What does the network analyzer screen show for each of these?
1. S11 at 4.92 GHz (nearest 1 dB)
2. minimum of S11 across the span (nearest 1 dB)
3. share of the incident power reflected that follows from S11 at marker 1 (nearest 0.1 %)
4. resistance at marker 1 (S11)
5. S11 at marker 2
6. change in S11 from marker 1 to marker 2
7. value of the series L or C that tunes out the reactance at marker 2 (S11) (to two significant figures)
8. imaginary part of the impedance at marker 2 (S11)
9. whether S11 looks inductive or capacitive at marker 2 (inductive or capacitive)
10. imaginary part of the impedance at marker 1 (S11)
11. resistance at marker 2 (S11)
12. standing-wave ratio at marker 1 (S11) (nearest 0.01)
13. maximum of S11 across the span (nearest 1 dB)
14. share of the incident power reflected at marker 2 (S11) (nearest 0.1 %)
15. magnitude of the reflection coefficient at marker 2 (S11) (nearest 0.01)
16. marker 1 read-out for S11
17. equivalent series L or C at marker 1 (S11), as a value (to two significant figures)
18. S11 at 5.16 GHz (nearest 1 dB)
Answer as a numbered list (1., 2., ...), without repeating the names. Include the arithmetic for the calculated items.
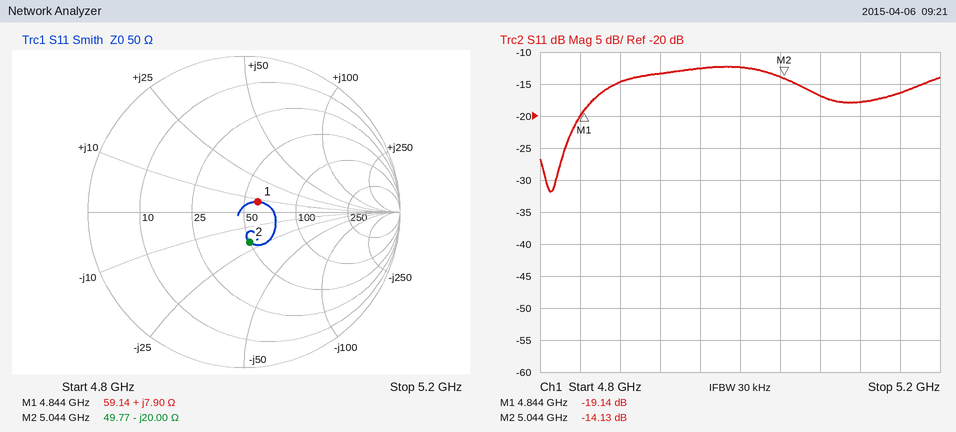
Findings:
1. -13 dB
2. -32 dB
3. 10^(-19.14/10) ≈ 1.2 %
4. 59.14 Ω
5. -14.13 dB
6. -14.13 − (-19.14) = 5.01 dB
7. L = 20 Ω/(2π × 5.044 GHz) ≈ 631 pH, so 630 pH to two significant figures
8. -20.00 Ω
9. capacitive
10. +7.90 Ω
11. 49.77 Ω
12. 1.25
13. -12 dB
14. 10^(-14.13/10) ≈ 3.9 %
15. 0.20
16. -19.14 dB
17. L = 7.9 Ω/(2π × 4.844 GHz) ≈ 260 pH
18. -16 dB
